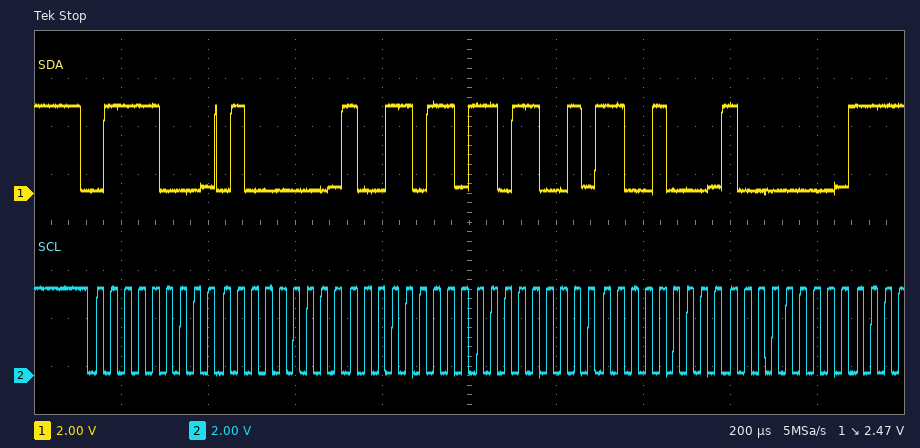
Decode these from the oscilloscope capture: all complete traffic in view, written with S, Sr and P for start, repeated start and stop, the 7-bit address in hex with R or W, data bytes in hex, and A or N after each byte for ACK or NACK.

S 3CW A 40 A 9B A D9 A C8 A 80 A
